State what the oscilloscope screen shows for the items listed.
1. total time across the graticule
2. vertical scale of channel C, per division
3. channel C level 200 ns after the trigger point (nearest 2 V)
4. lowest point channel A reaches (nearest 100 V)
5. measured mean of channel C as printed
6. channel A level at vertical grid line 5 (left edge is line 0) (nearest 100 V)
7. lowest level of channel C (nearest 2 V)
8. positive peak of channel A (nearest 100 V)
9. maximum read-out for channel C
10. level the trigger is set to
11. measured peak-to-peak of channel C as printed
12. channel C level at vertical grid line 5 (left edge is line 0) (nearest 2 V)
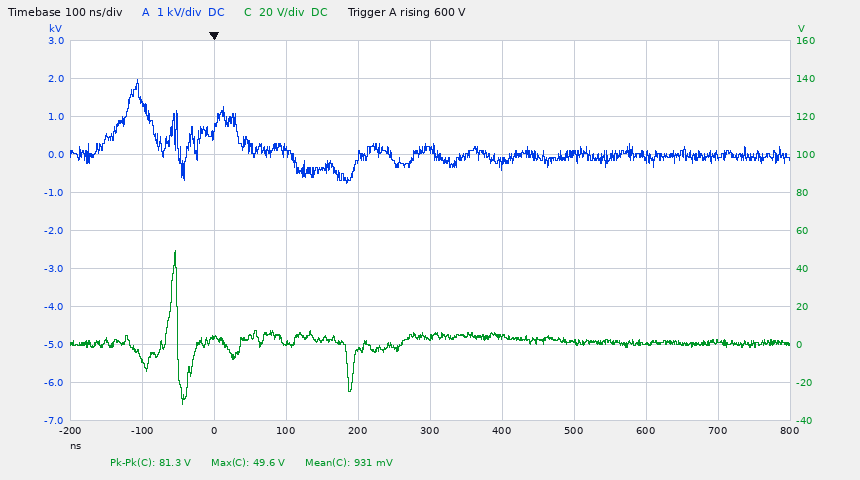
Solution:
1 µs
20 V
-4 V
-800 V
931 mV
100 V
-32 V
2.0 kV
49.6 V
600 V
81.3 V
4 V
